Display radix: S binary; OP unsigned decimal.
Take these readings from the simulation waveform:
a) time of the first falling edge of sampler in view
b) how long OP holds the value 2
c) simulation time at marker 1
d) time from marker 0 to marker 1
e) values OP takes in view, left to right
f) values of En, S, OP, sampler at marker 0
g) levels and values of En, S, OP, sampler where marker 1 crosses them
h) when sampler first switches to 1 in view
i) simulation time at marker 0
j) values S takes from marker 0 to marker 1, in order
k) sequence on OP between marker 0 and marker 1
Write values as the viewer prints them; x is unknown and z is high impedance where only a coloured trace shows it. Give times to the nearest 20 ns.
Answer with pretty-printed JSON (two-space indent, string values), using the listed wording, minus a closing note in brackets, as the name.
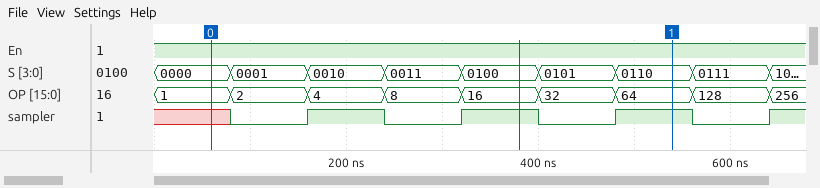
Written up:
{
  "time of the first falling edge of sampler in view": "240 ns",
  "how long OP holds the value 2": "80 ns",
  "simulation time at marker 1": "540 ns",
  "time from marker 0 to marker 1": "480 ns",
  "values OP takes in view, left to right": "1, 2, 4, 8, 16, 32, 64, 128, 256",
  "values of En, S, OP, sampler at marker 0": "En=1, S=0000, OP=1, sampler=x",
  "levels and values of En, S, OP, sampler where marker 1 crosses them": "En=1, S=0110, OP=64, sampler=1",
  "when sampler first switches to 1 in view": "160 ns",
  "simulation time at marker 0": "60 ns",
  "values S takes from marker 0 to marker 1, in order": "0000, 0001, 0010, 0011, 0100, 0101, 0110",
  "sequence on OP between marker 0 and marker 1": "1, 2, 4, 8, 16, 32, 64"
}
